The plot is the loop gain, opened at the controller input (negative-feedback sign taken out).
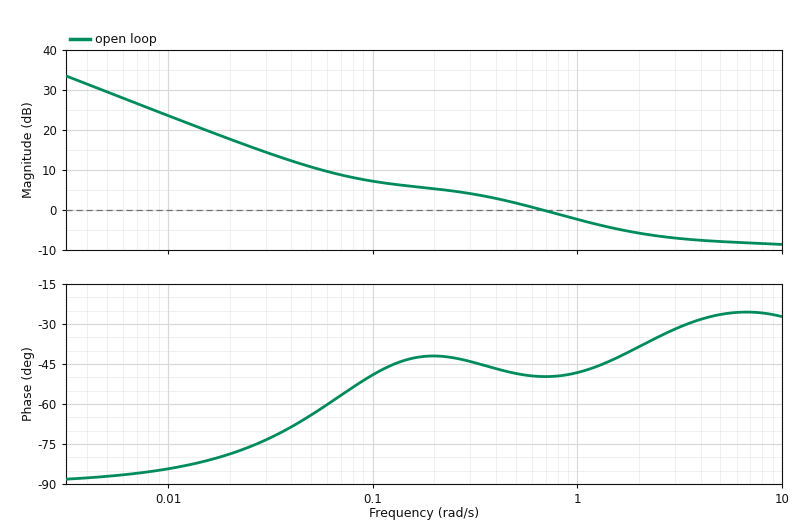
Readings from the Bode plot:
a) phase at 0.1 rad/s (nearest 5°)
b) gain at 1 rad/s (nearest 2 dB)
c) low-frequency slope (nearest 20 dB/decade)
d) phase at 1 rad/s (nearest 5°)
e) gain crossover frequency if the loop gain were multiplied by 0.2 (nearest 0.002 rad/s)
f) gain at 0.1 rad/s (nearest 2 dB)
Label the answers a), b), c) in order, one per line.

a) -50°
b) -2 dB
c) -20 dB/decade
d) -50°
e) 0.032 rad/s
f) 8 dB
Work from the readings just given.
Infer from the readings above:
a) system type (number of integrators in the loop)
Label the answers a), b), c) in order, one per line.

a) 1
